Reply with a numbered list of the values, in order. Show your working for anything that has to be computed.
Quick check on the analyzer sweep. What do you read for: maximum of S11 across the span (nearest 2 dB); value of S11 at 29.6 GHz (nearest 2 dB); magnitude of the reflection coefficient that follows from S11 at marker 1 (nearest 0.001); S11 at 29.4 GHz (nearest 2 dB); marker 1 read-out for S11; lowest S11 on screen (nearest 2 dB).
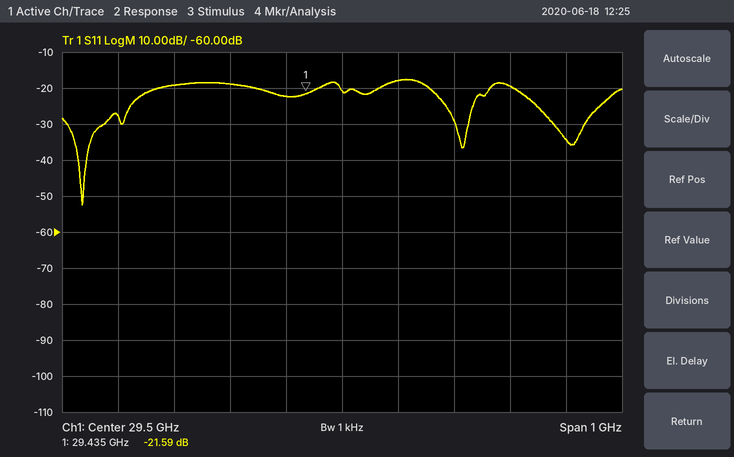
1. -18 dB
2. -18 dB
3. 10^(-21.59/20) ≈ 0.083
4. -22 dB
5. -21.59 dB
6. -52 dB
